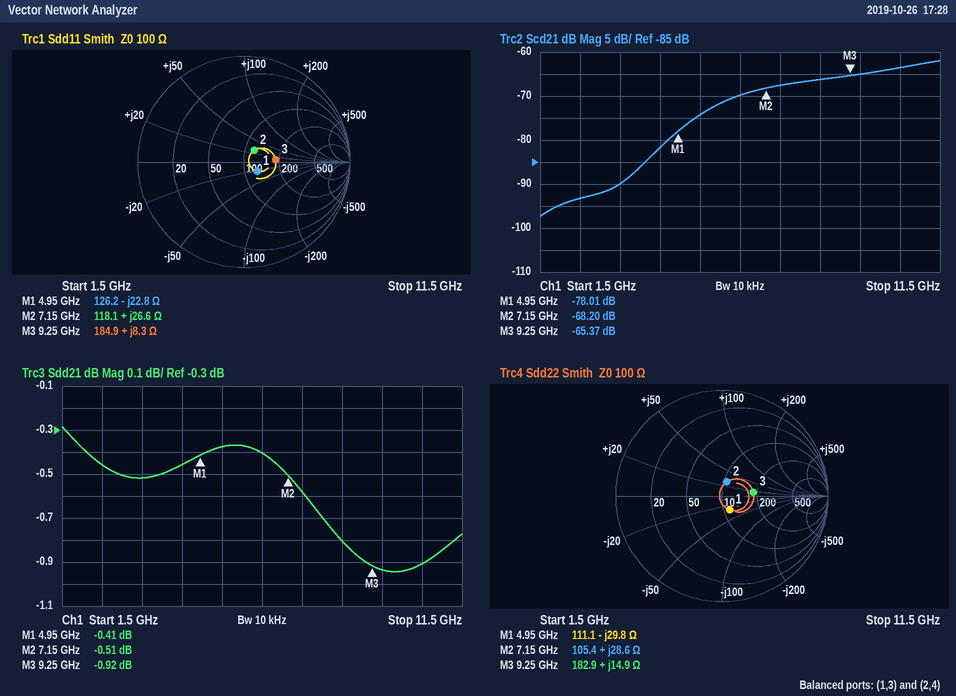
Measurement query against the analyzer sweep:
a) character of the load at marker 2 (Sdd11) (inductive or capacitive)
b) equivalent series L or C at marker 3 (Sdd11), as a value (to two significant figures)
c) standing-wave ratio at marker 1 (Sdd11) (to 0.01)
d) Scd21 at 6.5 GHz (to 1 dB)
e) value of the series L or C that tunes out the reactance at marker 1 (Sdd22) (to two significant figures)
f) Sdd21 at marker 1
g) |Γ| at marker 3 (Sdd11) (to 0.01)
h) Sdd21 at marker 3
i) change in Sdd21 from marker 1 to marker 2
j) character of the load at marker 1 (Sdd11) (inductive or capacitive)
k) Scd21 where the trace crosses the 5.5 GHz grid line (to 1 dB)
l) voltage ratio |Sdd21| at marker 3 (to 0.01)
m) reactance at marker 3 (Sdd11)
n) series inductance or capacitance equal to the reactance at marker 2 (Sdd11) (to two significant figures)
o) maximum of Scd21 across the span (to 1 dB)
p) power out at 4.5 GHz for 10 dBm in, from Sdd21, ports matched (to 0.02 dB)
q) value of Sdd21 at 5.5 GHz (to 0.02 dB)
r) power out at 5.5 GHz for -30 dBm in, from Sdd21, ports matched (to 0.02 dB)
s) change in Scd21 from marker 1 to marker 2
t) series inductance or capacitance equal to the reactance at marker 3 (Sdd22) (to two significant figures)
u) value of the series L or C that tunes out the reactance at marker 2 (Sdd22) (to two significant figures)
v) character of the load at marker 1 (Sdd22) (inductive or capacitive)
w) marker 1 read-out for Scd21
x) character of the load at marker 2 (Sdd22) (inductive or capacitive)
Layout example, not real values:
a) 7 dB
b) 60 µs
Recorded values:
a) inductive
b) 140 pH
c) 1.36
d) -70 dB
e) 960 pH
f) -0.41 dB
g) 0.30
h) -0.92 dB
i) -0.10 dB
j) capacitive
k) -74 dB
l) 0.90
m) +8.3 Ω
n) 590 pH
o) -62 dB
p) 9.54 dBm
q) -0.38 dB
r) -30.38 dBm
s) 9.81 dB
t) 260 pH
u) 780 fF
v) capacitive
w) -78.01 dB
x) inductive
